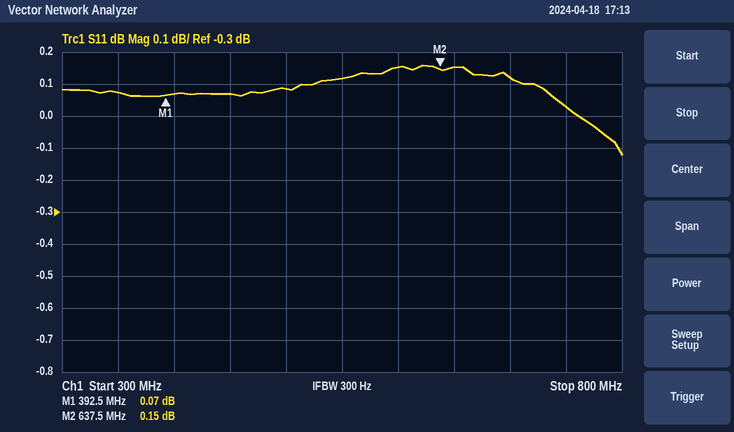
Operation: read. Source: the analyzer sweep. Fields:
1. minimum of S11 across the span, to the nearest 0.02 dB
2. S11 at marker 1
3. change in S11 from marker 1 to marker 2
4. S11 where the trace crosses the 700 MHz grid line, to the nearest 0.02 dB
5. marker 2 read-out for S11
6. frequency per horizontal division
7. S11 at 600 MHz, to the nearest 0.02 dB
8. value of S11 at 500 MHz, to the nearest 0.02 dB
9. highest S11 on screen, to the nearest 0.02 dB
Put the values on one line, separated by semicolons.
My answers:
-0.12 dB; 0.07 dB; 0.08 dB; 0.12 dB; 0.15 dB; 50 MHz; 0.16 dB; 0.08 dB; 0.16 dB
